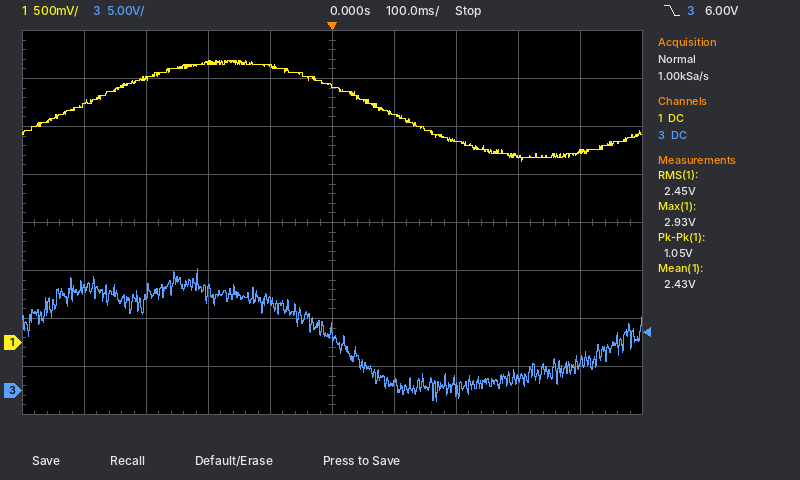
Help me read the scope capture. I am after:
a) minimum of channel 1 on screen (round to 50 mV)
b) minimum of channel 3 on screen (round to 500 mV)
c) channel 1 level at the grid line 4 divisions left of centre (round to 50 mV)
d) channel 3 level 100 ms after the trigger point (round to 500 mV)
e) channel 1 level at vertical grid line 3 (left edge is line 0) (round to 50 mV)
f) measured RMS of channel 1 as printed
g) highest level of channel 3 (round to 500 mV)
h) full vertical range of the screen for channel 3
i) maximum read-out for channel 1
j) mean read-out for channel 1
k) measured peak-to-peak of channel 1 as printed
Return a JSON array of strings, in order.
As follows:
["1.90 V", "-1.0 V", "2.50 V", "1.0 V", "2.90 V", "2.45 V", "12.5 V", "40 V", "2.93 V", "2.43 V", "1.05 V"]
